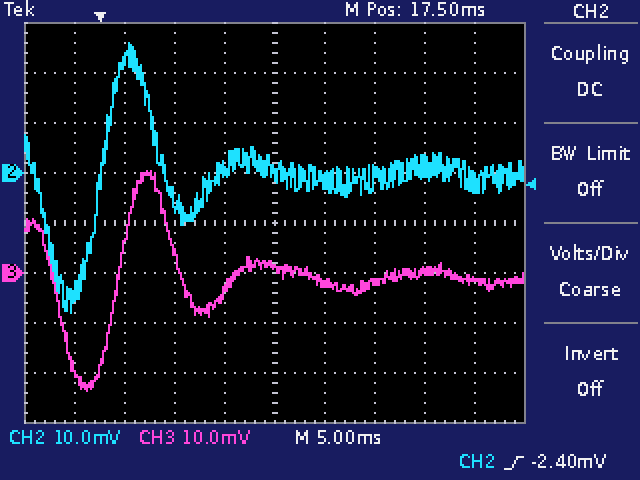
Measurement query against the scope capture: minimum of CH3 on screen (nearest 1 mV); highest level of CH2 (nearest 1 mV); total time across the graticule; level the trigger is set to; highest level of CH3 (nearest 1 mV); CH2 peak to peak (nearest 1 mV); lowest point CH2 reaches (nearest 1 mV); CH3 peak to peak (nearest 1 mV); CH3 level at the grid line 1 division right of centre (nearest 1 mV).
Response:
-24 mV
26 mV
50 ms
-2.40 mV
20 mV
54 mV
-28 mV
44 mV
-2 mV
